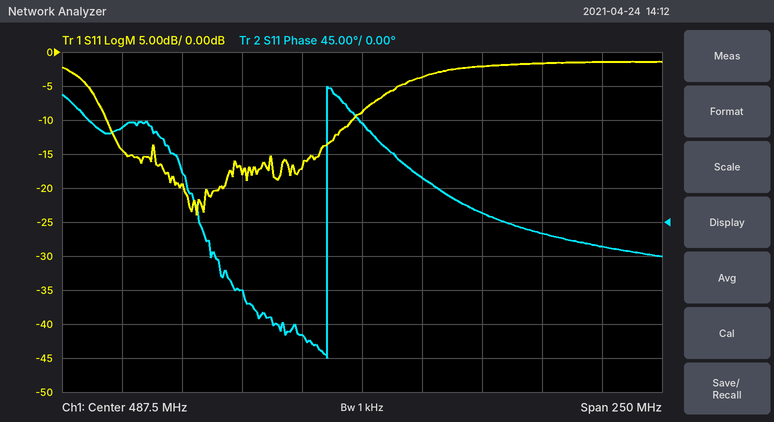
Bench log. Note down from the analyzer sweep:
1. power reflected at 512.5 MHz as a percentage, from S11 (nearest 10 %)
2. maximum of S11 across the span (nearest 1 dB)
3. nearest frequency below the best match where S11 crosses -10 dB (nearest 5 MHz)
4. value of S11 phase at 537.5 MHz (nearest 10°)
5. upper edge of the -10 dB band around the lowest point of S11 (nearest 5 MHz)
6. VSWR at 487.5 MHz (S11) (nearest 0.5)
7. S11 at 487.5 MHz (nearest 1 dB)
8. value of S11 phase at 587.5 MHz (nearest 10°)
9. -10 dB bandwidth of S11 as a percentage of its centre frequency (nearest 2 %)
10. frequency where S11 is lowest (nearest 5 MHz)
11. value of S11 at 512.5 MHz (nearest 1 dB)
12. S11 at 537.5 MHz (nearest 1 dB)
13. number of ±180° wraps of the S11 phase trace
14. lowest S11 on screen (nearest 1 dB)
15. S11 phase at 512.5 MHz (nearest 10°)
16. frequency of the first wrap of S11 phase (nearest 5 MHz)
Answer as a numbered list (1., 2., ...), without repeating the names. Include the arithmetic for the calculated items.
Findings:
1. 10^(-4/10) ≈ 40 %
2. -1 dB
3. 380 MHz
4. 10°
5. 485 MHz
6. |Γ| = 10^(-9/20) = 0.3548; VSWR = (1 + 0.3548)/(1 − 0.3548) ≈ 2.10, so 2.0 to the nearest 0.5
7. -9 dB
8. -30°
9. 105 MHz / 432.5 MHz ≈ 24 %
10. 420 MHz
11. -4 dB
12. -2 dB
13. 1
14. -24 dB
15. 60°
16. 475 MHz
